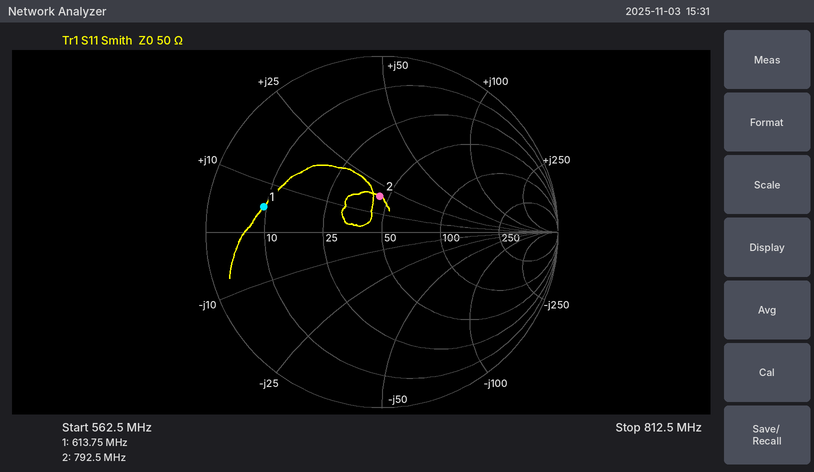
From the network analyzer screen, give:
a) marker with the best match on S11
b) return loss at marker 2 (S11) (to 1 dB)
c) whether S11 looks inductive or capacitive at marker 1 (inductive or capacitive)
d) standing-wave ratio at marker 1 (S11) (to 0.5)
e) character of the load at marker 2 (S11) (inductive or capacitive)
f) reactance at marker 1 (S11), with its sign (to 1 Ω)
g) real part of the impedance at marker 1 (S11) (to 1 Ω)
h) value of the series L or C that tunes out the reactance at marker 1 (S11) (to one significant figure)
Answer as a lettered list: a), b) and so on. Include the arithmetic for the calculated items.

a) marker 2
b) 14 dB
c) inductive
d) 5.5
e) inductive
f) +5 Ω
g) 9 Ω
h) C = 1/(2π × 613.75 MHz × 5 Ω) ≈ 51.9 pF, so 50 pF to one significant figure
